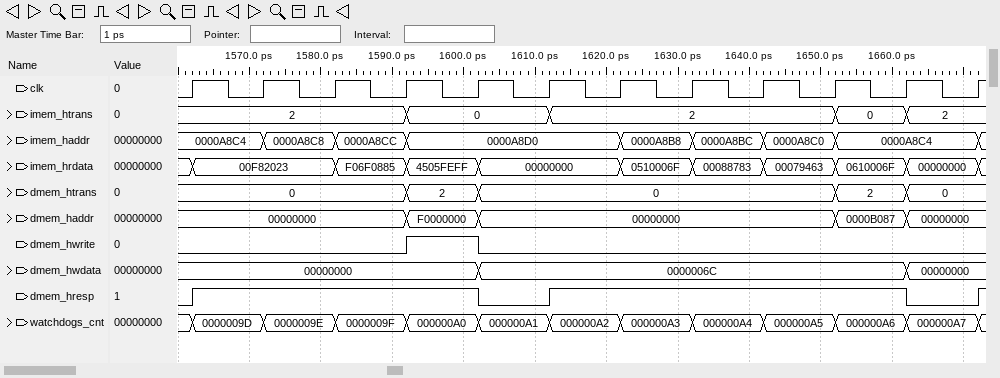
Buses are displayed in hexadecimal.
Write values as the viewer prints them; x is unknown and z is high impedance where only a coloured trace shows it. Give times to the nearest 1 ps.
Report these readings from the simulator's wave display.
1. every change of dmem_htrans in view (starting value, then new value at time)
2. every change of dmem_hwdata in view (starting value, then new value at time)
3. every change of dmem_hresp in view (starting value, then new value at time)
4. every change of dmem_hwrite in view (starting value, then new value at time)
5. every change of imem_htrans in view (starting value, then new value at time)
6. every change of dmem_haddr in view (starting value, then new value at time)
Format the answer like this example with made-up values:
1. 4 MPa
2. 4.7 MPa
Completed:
1. 0, 2 at 1592 ps, 0 at 1602 ps, 2 at 1652 ps, 0 at 1662 ps
2. 00000000, 0000006C at 1602 ps, 00000000 at 1662 ps
3. 0, 1 at 1562 ps, 0 at 1602 ps, 1 at 1612 ps, 0 at 1662 ps, 1 at 1672 ps
4. 0, 1 at 1592 ps, 0 at 1602 ps
5. 2, 0 at 1592 ps, 2 at 1612 ps, 0 at 1652 ps, 2 at 1662 ps
6. 00000000, F0000000 at 1592 ps, 00000000 at 1602 ps, 0000B087 at 1652 ps, 00000000 at 1662 ps
